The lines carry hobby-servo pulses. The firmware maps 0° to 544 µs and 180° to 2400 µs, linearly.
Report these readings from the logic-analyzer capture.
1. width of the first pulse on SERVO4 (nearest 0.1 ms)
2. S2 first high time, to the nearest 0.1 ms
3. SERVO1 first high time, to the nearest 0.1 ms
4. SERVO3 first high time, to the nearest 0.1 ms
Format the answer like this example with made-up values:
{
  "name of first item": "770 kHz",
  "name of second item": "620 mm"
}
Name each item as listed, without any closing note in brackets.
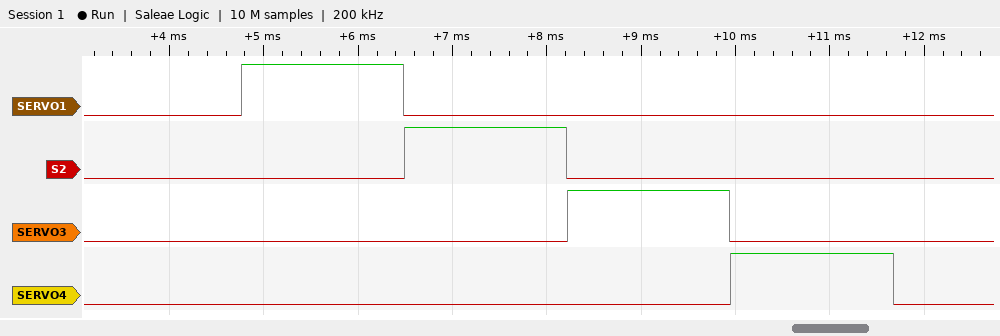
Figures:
{
  "width of the first pulse on SERVO4": "1.7 ms",
  "S2 first high time, to the nearest 0.1 ms": "1.7 ms",
  "SERVO1 first high time, to the nearest 0.1 ms": "1.7 ms",
  "SERVO3 first high time, to the nearest 0.1 ms": "1.7 ms"
}
